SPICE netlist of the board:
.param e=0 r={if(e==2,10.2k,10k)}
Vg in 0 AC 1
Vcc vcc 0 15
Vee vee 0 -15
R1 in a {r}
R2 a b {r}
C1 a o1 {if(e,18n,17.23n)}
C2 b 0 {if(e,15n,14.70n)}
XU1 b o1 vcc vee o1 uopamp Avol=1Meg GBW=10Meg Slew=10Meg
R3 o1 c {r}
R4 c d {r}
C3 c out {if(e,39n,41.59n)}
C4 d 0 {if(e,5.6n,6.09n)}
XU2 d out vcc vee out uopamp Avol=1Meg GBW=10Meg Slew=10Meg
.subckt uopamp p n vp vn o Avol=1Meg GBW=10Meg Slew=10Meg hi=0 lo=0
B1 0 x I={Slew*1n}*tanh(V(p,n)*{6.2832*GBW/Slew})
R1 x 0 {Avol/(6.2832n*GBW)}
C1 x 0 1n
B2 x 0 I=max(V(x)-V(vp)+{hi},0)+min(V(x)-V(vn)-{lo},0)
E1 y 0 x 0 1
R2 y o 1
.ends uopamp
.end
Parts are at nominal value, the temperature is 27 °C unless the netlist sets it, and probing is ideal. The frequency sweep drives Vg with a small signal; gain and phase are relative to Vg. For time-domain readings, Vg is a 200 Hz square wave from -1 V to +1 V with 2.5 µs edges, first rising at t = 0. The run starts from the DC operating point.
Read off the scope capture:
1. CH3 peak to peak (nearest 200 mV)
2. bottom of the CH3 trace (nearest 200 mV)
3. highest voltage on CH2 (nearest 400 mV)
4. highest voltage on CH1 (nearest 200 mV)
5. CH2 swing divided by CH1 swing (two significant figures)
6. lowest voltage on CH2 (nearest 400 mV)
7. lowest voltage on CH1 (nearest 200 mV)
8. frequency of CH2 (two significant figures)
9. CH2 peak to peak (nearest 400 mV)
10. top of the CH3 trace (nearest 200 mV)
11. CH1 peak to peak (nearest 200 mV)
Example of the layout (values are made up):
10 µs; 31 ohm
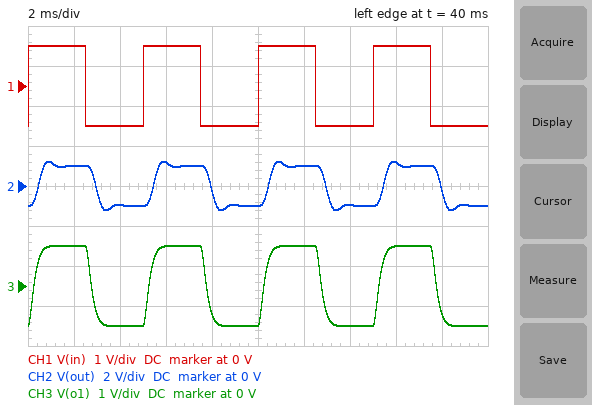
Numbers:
2.0 V; -1.0 V; 1.2 V; 1.0 V; 1.2; -1.2 V; -1.0 V; 200 Hz; 2.4 V; 1.0 V; 2.0 V
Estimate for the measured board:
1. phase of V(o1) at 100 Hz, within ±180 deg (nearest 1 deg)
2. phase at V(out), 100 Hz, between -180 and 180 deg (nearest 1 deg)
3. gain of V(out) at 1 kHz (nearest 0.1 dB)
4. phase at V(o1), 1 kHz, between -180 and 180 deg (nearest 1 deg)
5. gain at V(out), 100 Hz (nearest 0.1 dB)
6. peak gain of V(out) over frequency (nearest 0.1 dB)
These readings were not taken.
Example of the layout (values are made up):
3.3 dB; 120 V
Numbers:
-11 deg; -15 deg; -3.0 dB; -90 deg; 0 dB; 0 dB
